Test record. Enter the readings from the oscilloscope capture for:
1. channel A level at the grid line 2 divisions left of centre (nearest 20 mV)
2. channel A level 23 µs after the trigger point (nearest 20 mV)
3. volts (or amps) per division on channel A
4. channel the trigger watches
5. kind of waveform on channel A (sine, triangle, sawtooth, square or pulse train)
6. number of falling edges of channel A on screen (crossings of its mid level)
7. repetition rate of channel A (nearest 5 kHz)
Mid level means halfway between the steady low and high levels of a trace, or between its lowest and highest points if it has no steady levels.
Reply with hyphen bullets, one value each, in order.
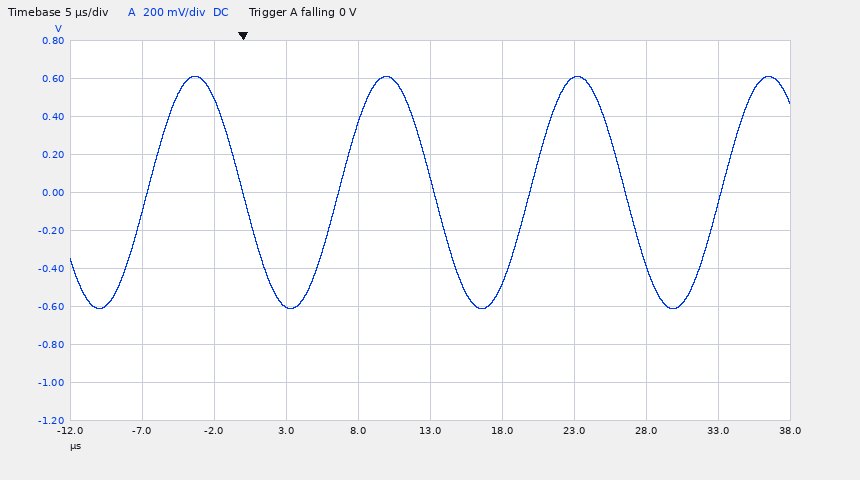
- -600 mV
- 600 mV
- 200 mV
- channel A
- sine
- 3
- 75 kHz
